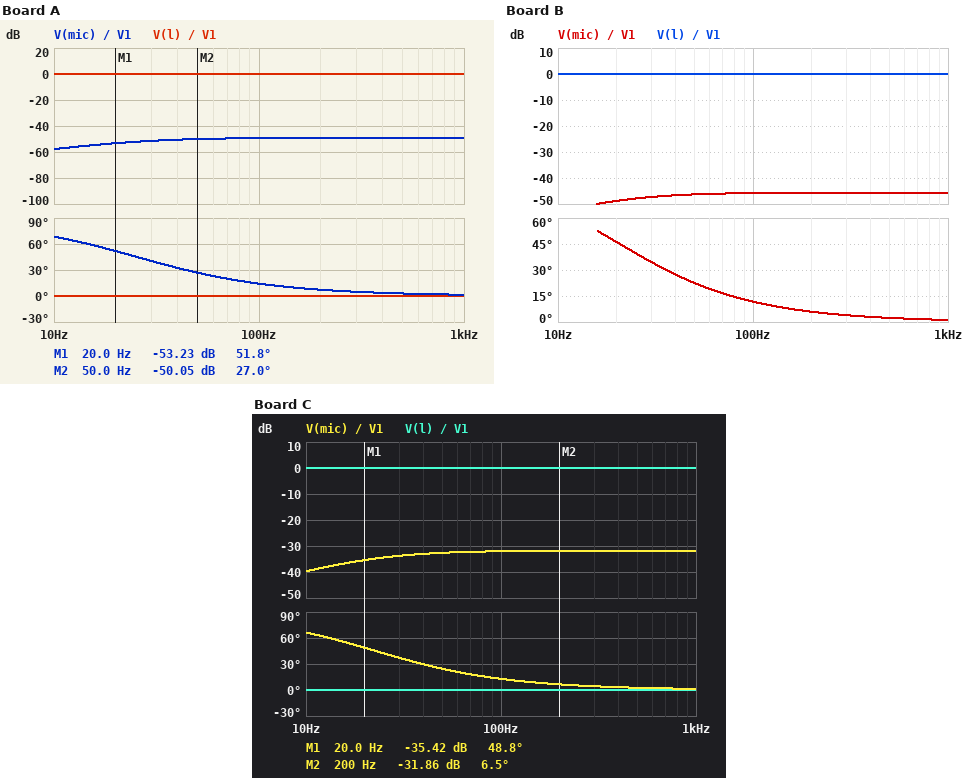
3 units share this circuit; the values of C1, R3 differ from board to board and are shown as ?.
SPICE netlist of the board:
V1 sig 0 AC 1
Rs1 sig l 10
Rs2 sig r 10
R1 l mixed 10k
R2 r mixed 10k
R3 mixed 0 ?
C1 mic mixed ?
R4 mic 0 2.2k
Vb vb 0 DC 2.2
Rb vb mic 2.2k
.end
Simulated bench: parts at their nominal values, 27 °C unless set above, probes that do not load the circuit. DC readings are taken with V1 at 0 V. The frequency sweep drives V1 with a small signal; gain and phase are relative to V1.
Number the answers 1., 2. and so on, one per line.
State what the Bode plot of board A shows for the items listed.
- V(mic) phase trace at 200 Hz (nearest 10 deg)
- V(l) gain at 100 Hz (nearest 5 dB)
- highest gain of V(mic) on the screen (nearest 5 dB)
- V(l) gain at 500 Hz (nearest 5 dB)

1. 10 deg
2. 0 dB
3. -50 dB
4. 0 dB
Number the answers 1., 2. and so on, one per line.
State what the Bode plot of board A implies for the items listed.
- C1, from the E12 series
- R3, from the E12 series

1. 5.6 µF
2. 18 Ω
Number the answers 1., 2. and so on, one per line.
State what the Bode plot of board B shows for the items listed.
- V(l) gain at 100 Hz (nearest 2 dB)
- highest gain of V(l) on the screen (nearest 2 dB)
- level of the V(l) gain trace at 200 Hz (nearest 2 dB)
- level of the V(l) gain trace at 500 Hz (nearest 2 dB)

1. 0 dB
2. 0 dB
3. 0 dB
4. 0 dB
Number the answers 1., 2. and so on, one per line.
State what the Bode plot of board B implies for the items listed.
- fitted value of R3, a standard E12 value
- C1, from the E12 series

1. 27 Ω
2. 6.8 µF
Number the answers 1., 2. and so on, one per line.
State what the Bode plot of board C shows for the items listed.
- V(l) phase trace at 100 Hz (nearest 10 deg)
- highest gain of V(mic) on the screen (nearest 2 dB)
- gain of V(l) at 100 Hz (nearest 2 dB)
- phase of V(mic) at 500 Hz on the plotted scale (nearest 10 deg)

1. 0 deg
2. -32 dB
3. 0 dB
4. 0 deg
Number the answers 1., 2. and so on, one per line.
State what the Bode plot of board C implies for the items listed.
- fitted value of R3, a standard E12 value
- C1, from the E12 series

1. 150 Ω
2. 5.6 µF
